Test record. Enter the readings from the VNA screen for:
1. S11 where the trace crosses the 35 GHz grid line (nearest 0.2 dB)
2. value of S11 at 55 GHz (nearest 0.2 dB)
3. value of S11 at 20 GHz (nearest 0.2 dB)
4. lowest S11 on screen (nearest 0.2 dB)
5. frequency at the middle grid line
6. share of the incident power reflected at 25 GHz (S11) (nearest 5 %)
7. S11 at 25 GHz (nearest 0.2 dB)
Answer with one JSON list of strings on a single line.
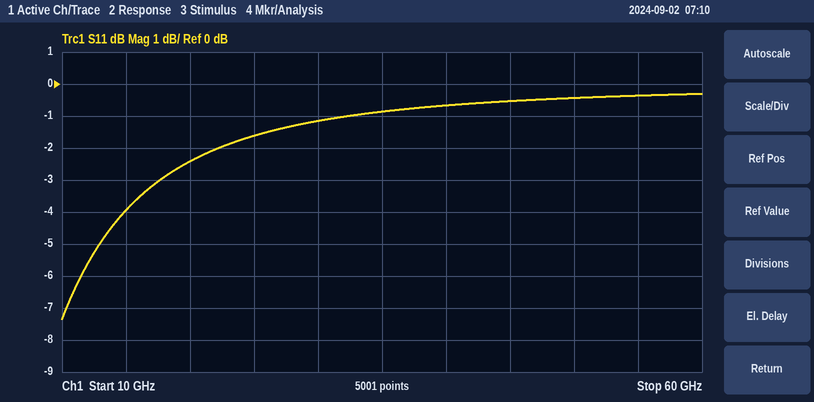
["-0.8 dB", "-0.4 dB", "-2.4 dB", "-7.4 dB", "35 GHz", "70 %", "-1.6 dB"]
